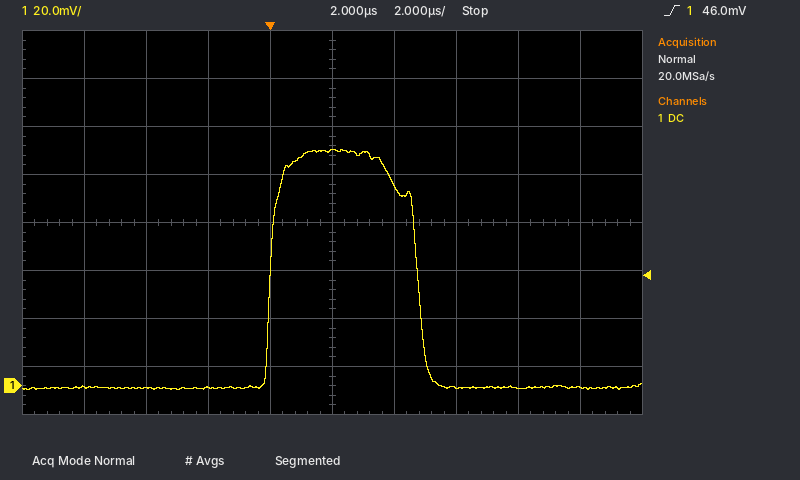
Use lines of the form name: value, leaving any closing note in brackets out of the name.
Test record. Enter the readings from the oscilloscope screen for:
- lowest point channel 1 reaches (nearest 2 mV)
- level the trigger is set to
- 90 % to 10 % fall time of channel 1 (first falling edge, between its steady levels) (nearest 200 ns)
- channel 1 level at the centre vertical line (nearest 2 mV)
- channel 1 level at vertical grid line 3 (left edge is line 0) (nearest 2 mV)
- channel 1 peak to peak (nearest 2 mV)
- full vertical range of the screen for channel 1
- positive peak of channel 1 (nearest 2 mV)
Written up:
lowest point channel 1 reaches: -2 mV
level the trigger is set to: 46.0 mV
90 % to 10 % fall time of channel 1 (first falling edge, between its steady levels): 1.2 µs
channel 1 level at the centre vertical line: 98 mV
channel 1 level at vertical grid line 3 (left edge is line 0): 0 mV
channel 1 peak to peak: 100 mV
full vertical range of the screen for channel 1: 160 mV
positive peak of channel 1: 98 mV
